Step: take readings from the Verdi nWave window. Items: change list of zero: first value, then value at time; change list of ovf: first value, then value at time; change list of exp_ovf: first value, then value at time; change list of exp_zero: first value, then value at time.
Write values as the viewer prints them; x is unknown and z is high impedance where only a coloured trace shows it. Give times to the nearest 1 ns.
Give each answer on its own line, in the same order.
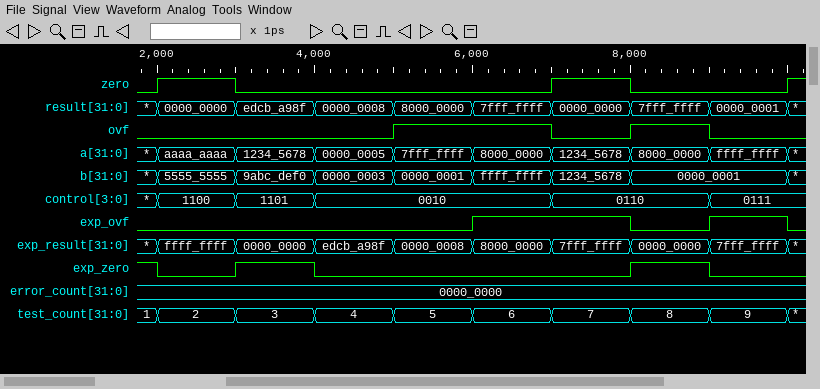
0, 1 at 2 ns, 0 at 3 ns, 1 at 7 ns, 0 at 8 ns, 1 at 10 ns
0, 1 at 5 ns, 0 at 7 ns, 1 at 8 ns, 0 at 9 ns
0, 1 at 6 ns, 0 at 8 ns, 1 at 9 ns, 0 at 10 ns
1, 0 at 2 ns, 1 at 3 ns, 0 at 4 ns, 1 at 8 ns, 0 at 9 ns
